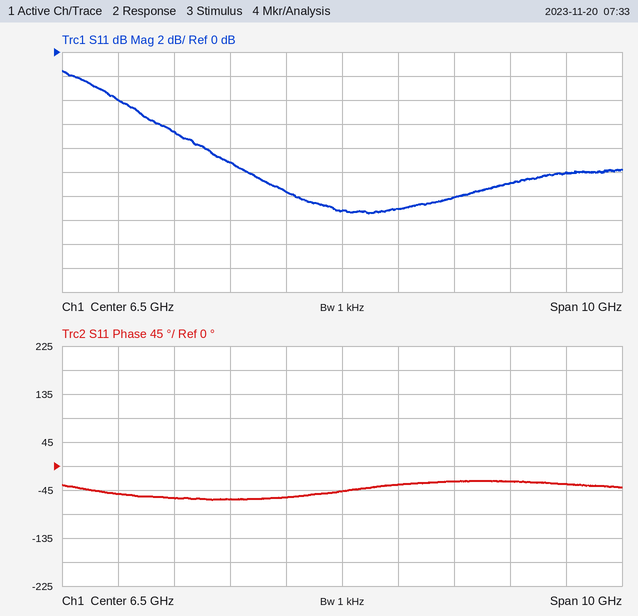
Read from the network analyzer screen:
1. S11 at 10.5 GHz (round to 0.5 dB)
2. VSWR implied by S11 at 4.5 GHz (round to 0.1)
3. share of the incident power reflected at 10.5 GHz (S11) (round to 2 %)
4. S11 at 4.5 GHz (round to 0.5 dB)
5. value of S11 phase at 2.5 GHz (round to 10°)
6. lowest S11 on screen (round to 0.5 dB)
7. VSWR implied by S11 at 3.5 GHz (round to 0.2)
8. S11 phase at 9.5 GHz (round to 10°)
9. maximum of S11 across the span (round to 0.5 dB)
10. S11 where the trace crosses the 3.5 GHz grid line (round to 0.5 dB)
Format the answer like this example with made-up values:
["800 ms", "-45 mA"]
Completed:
["-10.0 dB", "2.1", "10 %", "-9.0 dB", "-50°", "-13.5 dB", "2.8", "-30°", "-1.5 dB", "-6.5 dB"]
